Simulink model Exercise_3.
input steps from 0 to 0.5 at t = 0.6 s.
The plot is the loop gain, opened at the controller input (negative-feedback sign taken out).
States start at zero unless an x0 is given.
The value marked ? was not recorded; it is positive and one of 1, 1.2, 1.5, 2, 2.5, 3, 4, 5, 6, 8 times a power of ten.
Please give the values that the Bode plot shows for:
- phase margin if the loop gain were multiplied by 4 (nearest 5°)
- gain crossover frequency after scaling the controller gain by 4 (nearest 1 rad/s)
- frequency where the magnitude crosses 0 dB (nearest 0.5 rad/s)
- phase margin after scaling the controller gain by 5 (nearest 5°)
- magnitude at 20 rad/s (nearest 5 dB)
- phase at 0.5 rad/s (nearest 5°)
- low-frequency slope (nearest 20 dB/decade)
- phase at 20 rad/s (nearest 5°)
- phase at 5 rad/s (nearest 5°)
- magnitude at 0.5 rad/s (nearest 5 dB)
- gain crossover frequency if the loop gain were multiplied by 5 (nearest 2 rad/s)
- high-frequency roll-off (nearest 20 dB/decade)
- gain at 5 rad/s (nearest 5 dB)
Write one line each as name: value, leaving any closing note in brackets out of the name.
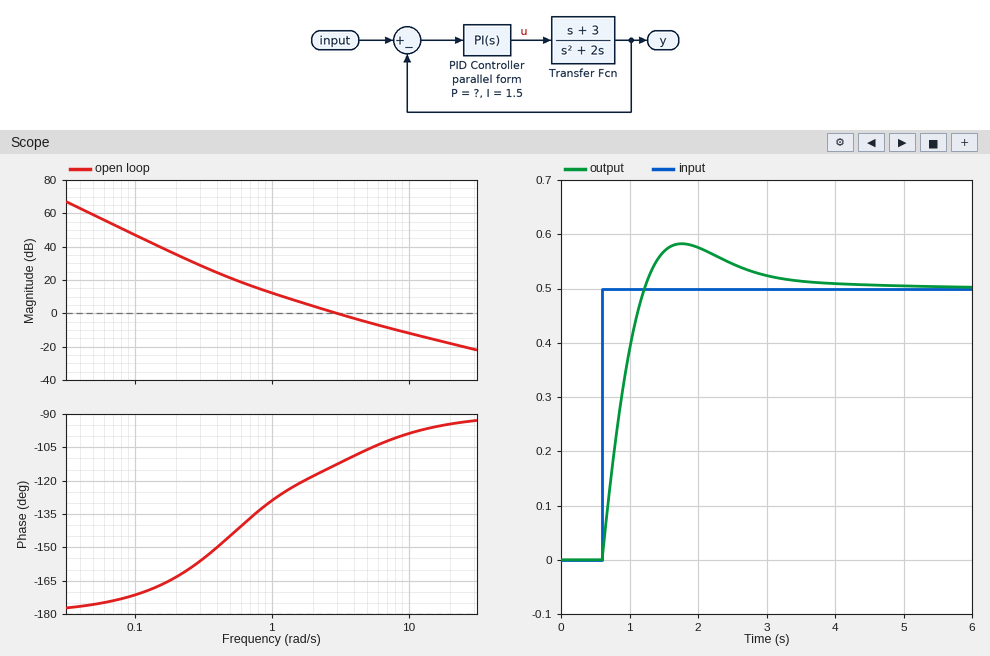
phase margin if the loop gain were multiplied by 4: 80°
gain crossover frequency after scaling the controller gain by 4: 10 rad/s
frequency where the magnitude crosses 0 dB: 3.0 rad/s
phase margin after scaling the controller gain by 5: 85°
magnitude at 20 rad/s: -20 dB
phase at 0.5 rad/s: -145°
low-frequency slope: -40 dB/decade
phase at 20 rad/s: -95°
phase at 5 rad/s: -105°
magnitude at 0.5 rad/s: 20 dB
gain crossover frequency if the loop gain were multiplied by 5: 12 rad/s
high-frequency roll-off: -20 dB/decade
gain at 5 rad/s: -5 dB
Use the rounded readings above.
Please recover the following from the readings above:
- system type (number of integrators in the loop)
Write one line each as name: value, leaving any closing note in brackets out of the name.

system type: 2
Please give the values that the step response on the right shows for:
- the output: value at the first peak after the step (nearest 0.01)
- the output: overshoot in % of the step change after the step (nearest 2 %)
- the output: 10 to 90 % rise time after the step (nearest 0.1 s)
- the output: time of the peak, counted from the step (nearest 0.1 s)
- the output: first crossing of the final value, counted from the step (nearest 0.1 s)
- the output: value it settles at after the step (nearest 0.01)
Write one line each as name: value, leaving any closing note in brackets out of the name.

the output: value at the first peak after the step: 0.58
the output: overshoot in % of the step change after the step: 16 %
the output: 10 to 90 % rise time after the step: 0.5 s
the output: time of the peak, counted from the step: 1.2 s
the output: first crossing of the final value, counted from the step: 0.6 s
the output: value it settles at after the step: 0.50
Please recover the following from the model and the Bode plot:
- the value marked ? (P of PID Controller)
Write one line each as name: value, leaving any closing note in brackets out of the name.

the value marked ?: 2.5
